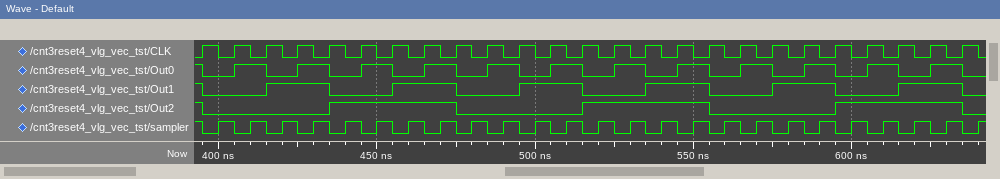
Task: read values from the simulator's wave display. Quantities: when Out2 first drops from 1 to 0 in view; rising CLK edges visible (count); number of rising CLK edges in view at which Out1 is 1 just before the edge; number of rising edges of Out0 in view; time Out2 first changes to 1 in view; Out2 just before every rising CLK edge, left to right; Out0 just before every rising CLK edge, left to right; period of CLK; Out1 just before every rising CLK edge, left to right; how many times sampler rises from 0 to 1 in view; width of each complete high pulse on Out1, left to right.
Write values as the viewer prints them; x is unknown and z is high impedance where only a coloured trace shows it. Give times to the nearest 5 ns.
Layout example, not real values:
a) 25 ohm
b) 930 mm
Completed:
a) 395 ns
b) 25
c) 13
d) 12
e) 435 ns
f) 1 0 0 0 0 1 1 1 1 0 0 0 0 1 1 1 1 0 0 0 0 1 1 1 1
g) 1 0 1 0 1 0 1 0 1 0 1 0 1 0 1 0 1 0 1 0 1 0 1 0 1
h) 10 ns
i) 1 0 0 1 1 0 0 1 1 0 0 1 1 0 0 1 1 0 0 1 1 0 0 1 1
j) 25
k) 20 ns, 20 ns, 20 ns, 20 ns, 20 ns, 20 ns
